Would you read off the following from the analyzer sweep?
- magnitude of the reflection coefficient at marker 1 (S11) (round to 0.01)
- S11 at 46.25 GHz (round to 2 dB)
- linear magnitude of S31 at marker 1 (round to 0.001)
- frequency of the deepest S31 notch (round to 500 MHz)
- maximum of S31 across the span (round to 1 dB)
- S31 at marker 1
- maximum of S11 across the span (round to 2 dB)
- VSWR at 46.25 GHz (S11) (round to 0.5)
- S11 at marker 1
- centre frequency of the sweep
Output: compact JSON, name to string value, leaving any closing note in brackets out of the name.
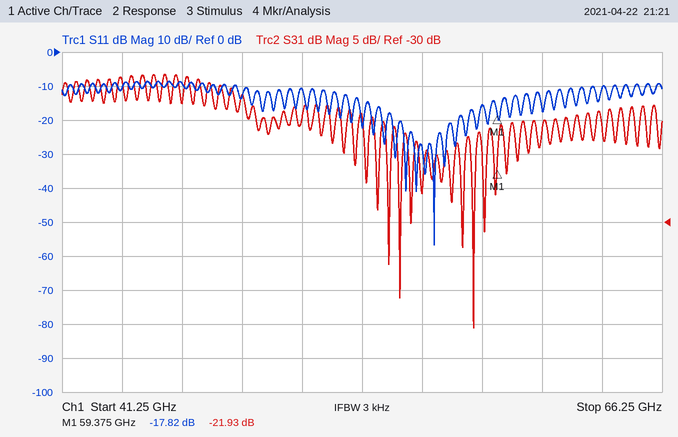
{"magnitude of the reflection coefficient at marker 1 (S11)": "0.13", "S11 at 46.25 GHz": "-10 dB", "linear magnitude of S31 at marker 1": "0.080", "frequency of the deepest S31 notch": "58.5 GHz", "maximum of S31 across the span": "-8 dB", "S31 at marker 1": "-21.93 dB", "maximum of S11 across the span": "-8 dB", "VSWR at 46.25 GHz (S11)": "2.0", "S11 at marker 1": "-17.82 dB", "centre frequency of the sweep": "53.75 GHz"}
